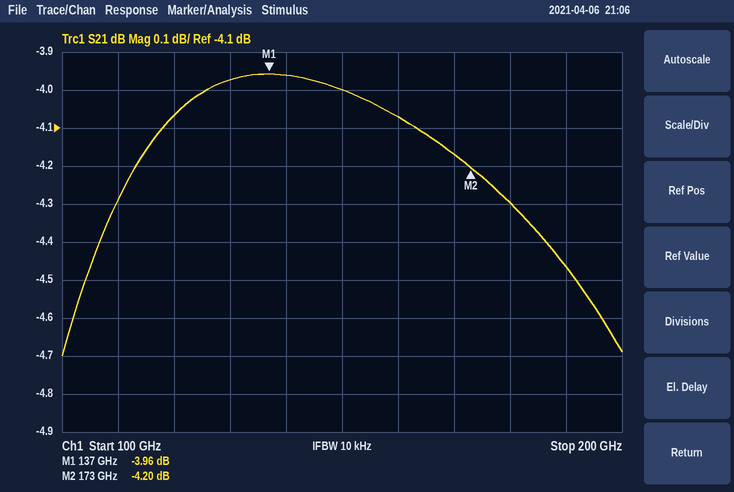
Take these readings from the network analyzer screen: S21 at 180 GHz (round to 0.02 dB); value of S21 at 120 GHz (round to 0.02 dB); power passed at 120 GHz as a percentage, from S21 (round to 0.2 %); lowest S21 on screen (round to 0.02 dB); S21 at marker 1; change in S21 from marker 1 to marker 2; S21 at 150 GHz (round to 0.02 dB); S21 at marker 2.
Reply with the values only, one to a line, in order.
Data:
-4.30 dB
-4.06 dB
39.2 %
-4.70 dB
-3.96 dB
-0.24 dB
-4.00 dB
-4.20 dB
